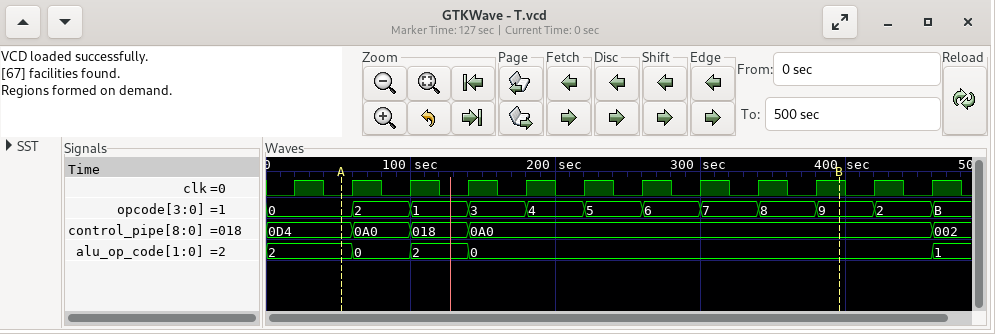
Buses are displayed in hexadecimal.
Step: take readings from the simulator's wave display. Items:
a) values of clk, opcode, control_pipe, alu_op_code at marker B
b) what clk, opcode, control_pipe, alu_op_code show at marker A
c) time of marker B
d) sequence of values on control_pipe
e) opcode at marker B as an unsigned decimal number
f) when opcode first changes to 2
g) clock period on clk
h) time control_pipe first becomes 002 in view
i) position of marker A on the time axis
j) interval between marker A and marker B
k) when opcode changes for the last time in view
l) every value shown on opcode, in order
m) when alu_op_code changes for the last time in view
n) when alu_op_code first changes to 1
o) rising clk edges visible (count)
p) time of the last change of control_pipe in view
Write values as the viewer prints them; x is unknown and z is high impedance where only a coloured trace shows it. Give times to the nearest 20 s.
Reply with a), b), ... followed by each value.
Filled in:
a) clk=1, opcode=9, control_pipe=0A0, alu_op_code=0
b) clk=0, opcode=0, control_pipe=0D4, alu_op_code=2
c) 400 s
d) 0D4, 0A0, 018, 0A0, 002
e) 9
f) 60 s
g) 40 s
h) 460 s
i) 60 s
j) 340 s
k) 460 s
l) 0, 2, 1, 3, 4, 5, 6, 7, 8, 9, 2, B
m) 460 s
n) 460 s
o) 12
p) 460 s
